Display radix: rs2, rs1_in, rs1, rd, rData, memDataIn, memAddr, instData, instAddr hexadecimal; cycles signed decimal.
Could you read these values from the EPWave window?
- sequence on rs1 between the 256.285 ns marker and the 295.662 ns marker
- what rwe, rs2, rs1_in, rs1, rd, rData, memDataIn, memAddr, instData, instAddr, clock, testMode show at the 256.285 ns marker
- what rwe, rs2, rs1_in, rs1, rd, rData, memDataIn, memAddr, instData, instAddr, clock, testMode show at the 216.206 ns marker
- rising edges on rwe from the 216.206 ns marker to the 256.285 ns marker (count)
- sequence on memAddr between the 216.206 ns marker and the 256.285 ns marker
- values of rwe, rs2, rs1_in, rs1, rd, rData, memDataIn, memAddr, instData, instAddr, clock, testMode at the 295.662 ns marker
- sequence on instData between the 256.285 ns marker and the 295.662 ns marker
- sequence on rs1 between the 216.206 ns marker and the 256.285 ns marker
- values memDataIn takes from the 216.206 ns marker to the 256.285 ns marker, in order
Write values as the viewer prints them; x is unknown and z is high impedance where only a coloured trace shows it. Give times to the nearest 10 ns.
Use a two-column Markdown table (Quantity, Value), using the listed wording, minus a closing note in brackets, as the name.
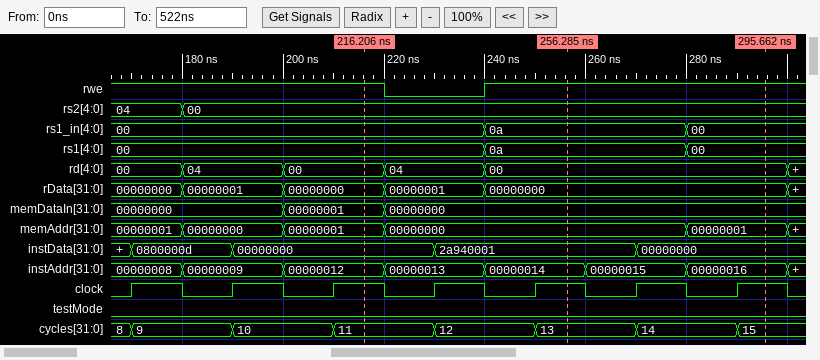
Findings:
| Quantity | Value |
|---|---|
| sequence on rs1 between the 256.285 ns marker and the 295.662 ns marker | 0a, 00 |
| what rwe, rs2, rs1_in, rs1, rd, rData, memDataIn, memAddr, instData, instAddr, clock, testMode show at the 256.285 ns marker | rwe=1, rs2=00, rs1_in=0a, rs1=0a, rd=00, rData=00000000, memDataIn=00000000, memAddr=00000000, instData=2a940001, instAddr=00000014, clock=1, testMode=0 |
| what rwe, rs2, rs1_in, rs1, rd, rData, memDataIn, memAddr, instData, instAddr, clock, testMode show at the 216.206 ns marker | rwe=1, rs2=00, rs1_in=00, rs1=00, rd=00, rData=00000000, memDataIn=00000001, memAddr=00000001, instData=00000000, instAddr=00000012, clock=1, testMode=0 |
| rising edges on rwe from the 216.206 ns marker to the 256.285 ns marker | 1 |
| sequence on memAddr between the 216.206 ns marker and the 256.285 ns marker | 00000001, 00000000 |
| values of rwe, rs2, rs1_in, rs1, rd, rData, memDataIn, memAddr, instData, instAddr, clock, testMode at the 295.662 ns marker | rwe=1, rs2=00, rs1_in=00, rs1=00, rd=00, rData=00000000, memDataIn=00000000, memAddr=00000001, instData=00000000, instAddr=00000016, clock=1, testMode=0 |
| sequence on instData between the 256.285 ns marker and the 295.662 ns marker | 2a940001, 00000000 |
| sequence on rs1 between the 216.206 ns marker and the 256.285 ns marker | 00, 0a |
| values memDataIn takes from the 216.206 ns marker to the 256.285 ns marker, in order | 00000001, 00000000 |
